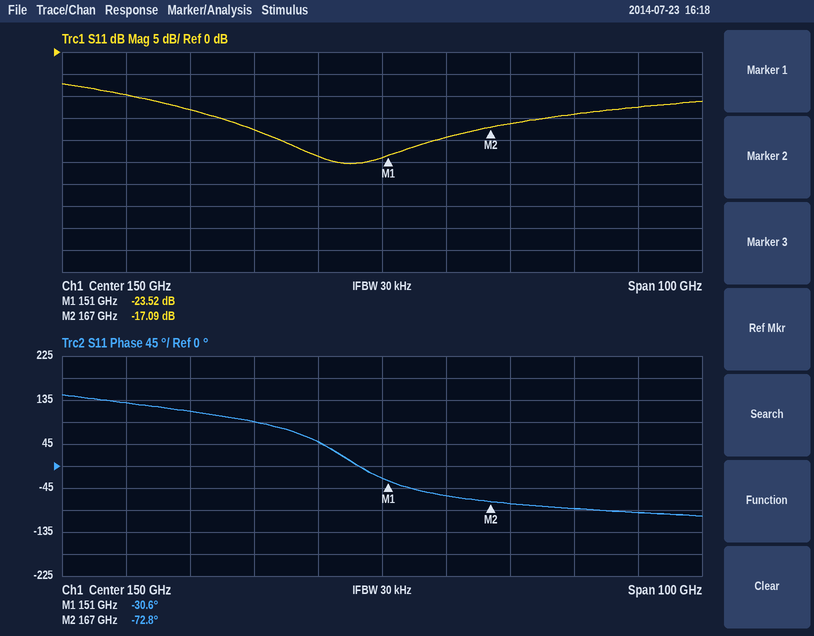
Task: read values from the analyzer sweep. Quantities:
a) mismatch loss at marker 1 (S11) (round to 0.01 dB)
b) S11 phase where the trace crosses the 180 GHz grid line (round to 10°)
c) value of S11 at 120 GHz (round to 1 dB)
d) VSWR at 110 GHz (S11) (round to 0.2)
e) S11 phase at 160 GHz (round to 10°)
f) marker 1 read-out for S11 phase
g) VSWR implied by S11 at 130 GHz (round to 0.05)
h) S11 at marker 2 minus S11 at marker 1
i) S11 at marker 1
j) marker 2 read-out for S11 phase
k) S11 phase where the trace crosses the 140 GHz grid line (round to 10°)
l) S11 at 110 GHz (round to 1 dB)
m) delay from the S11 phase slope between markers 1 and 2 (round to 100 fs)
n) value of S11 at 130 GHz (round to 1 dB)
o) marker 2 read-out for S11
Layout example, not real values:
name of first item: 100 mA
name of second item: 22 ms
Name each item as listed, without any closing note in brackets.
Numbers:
mismatch loss at marker 1 (S11): 0.02 dB
S11 phase where the trace crosses the 180 GHz grid line: -90°
value of S11 at 120 GHz: -13 dB
VSWR at 110 GHz (S11): 2.0
S11 phase at 160 GHz: -60°
marker 1 read-out for S11 phase: -30.6°
VSWR implied by S11 at 130 GHz: 1.30
S11 at marker 2 minus S11 at marker 1: 6.43 dB
S11 at marker 1: -23.52 dB
marker 2 read-out for S11 phase: -72.8°
S11 phase where the trace crosses the 140 GHz grid line: 50°
S11 at 110 GHz: -10 dB
delay from the S11 phase slope between markers 1 and 2: 7.3 ps
value of S11 at 130 GHz: -18 dB
marker 2 read-out for S11: -17.09 dB
